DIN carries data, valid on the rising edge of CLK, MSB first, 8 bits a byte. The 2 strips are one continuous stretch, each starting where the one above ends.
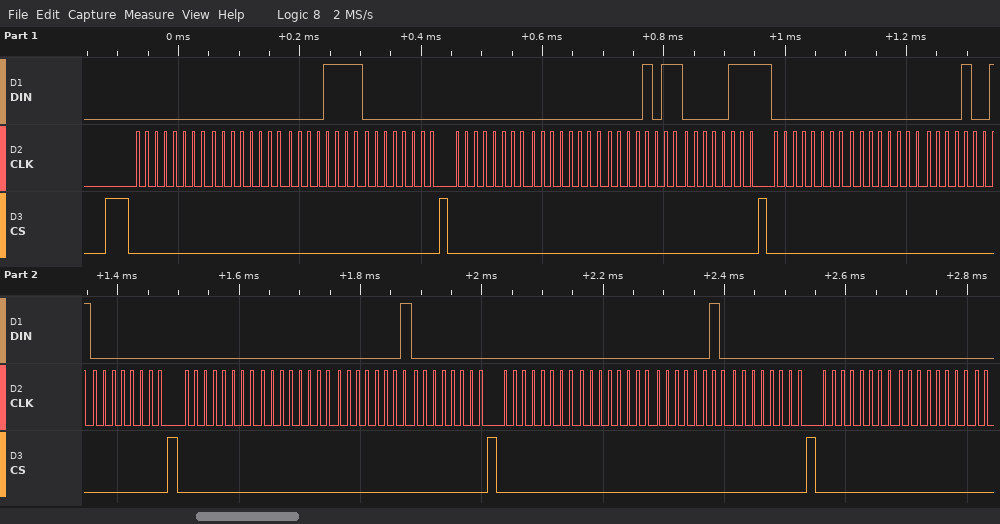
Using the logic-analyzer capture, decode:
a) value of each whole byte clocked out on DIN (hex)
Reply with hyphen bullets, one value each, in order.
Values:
- 0x00 0x00 0x0F 0x00 0x00 0x00 0x0B 0x07 0x00 0x00 0x09 0x00 0x00 0x00 0x01 0x00 0x00 0x00 0x02 0x00 0x00 0x00
